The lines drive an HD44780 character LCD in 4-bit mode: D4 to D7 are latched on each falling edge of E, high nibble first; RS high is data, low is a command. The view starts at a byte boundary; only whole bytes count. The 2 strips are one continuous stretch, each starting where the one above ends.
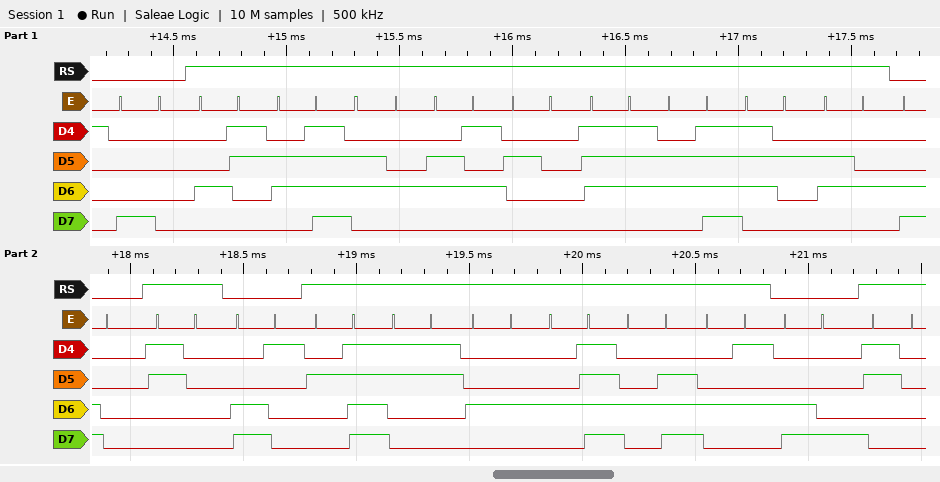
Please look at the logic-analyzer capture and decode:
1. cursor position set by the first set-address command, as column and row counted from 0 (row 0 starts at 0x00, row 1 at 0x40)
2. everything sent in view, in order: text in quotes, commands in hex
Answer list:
column 0, row 0
0x80 "Code word" 0xC0 "0" 0xC1 "/3DONE" 0xC8 "0"
